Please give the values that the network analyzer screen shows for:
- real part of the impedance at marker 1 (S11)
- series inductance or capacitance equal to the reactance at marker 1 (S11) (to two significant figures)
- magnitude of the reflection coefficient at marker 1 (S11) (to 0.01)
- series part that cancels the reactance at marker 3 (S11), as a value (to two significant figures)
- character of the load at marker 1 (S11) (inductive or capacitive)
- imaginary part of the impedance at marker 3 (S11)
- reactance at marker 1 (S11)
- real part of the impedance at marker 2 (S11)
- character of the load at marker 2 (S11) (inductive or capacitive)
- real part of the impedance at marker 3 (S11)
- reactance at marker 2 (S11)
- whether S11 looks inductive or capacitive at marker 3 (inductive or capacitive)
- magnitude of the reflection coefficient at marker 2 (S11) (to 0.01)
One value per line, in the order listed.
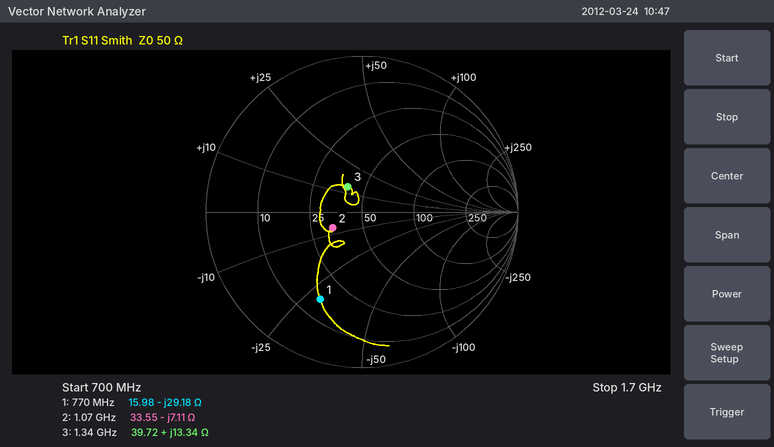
15.98 Ω
7.1 pF
0.62
8.9 pF
capacitive
+13.34 Ω
-29.18 Ω
33.55 Ω
capacitive
39.72 Ω
-7.11 Ω
inductive
0.21
